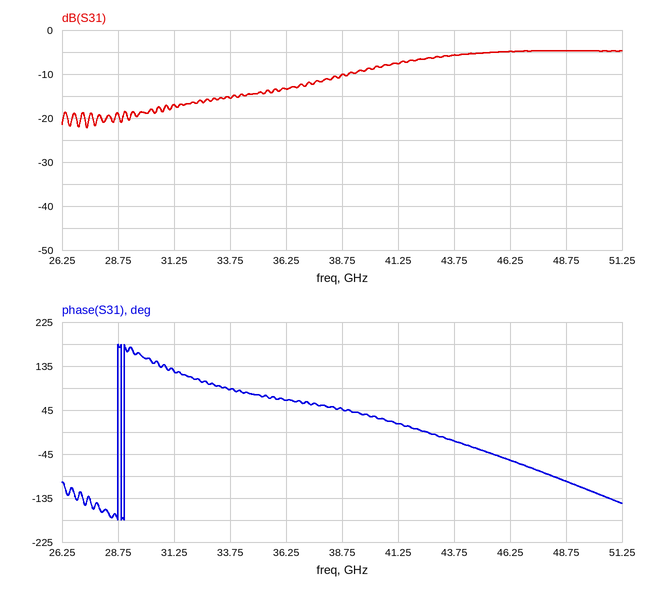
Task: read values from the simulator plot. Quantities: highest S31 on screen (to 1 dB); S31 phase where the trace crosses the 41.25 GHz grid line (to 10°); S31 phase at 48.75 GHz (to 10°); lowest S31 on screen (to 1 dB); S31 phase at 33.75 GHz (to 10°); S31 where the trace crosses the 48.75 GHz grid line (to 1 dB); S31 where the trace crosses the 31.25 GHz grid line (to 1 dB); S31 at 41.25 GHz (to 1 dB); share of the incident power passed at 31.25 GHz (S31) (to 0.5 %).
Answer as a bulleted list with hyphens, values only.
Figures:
- -5 dB
- 20°
- -100°
- -22 dB
- 90°
- -5 dB
- -17 dB
- -8 dB
- 2.0 %
